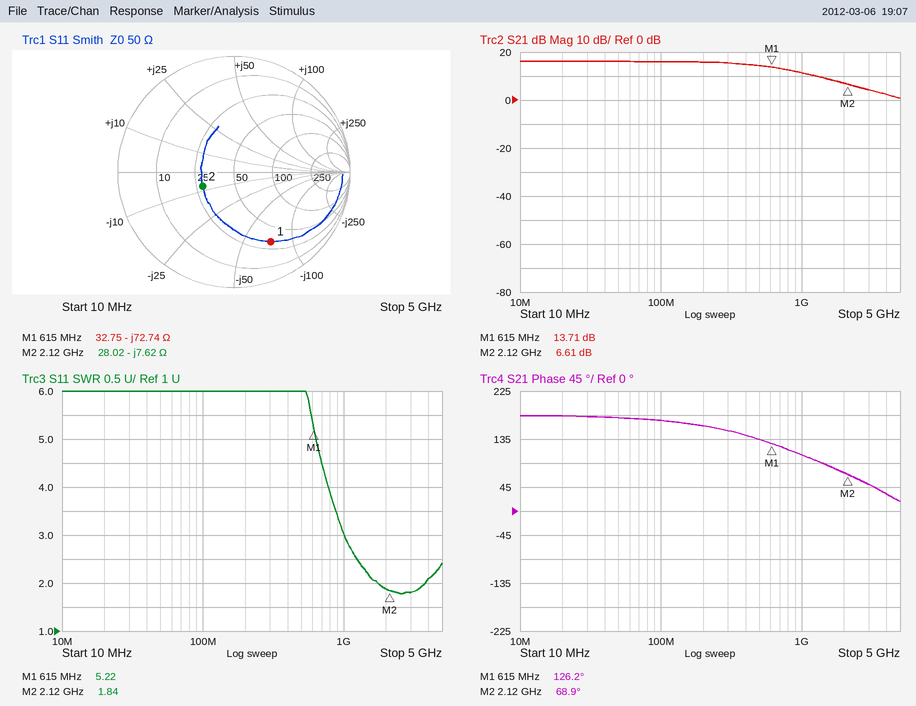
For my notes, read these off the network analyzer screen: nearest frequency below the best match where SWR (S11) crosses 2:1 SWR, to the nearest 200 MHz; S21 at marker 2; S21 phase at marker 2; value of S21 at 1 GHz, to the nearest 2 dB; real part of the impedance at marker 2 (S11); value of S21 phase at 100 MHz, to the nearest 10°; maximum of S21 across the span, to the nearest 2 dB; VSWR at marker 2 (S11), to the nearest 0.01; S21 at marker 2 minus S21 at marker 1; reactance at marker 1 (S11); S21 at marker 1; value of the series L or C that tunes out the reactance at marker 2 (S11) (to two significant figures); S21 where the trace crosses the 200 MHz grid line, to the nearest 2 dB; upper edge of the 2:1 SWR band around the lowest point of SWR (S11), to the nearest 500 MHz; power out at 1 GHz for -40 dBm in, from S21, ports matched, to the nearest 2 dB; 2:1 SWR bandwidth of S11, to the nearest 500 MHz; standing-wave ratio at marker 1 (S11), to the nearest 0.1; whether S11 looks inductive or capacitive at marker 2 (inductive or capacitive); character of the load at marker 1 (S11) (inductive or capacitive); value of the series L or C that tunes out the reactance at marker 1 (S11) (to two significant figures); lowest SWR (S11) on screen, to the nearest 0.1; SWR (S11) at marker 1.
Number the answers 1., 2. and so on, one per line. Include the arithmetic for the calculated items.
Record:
1. 1.8 GHz
2. 6.61 dB
3. 68.9°
4. 12 dB
5. 28.02 Ω
6. 170°
7. 16 dB
8. 1.84
9. 6.61 − (13.71) = -7.10 dB
10. -72.74 Ω
11. 13.71 dB
12. L = 7.62 Ω/(2π × 2.12 GHz) ≈ 572 pH, so 570 pH to two significant figures
13. 16 dB
14. 4.0 GHz
15. -40 dBm + (12 dB) = -28 dBm
16. 4.0 GHz − 1.8 GHz = 2.2 GHz
17. 5.2
18. capacitive
19. capacitive
20. L = 72.74 Ω/(2π × 615 MHz) ≈ 19 nH
21. 1.8
22. 5.22
